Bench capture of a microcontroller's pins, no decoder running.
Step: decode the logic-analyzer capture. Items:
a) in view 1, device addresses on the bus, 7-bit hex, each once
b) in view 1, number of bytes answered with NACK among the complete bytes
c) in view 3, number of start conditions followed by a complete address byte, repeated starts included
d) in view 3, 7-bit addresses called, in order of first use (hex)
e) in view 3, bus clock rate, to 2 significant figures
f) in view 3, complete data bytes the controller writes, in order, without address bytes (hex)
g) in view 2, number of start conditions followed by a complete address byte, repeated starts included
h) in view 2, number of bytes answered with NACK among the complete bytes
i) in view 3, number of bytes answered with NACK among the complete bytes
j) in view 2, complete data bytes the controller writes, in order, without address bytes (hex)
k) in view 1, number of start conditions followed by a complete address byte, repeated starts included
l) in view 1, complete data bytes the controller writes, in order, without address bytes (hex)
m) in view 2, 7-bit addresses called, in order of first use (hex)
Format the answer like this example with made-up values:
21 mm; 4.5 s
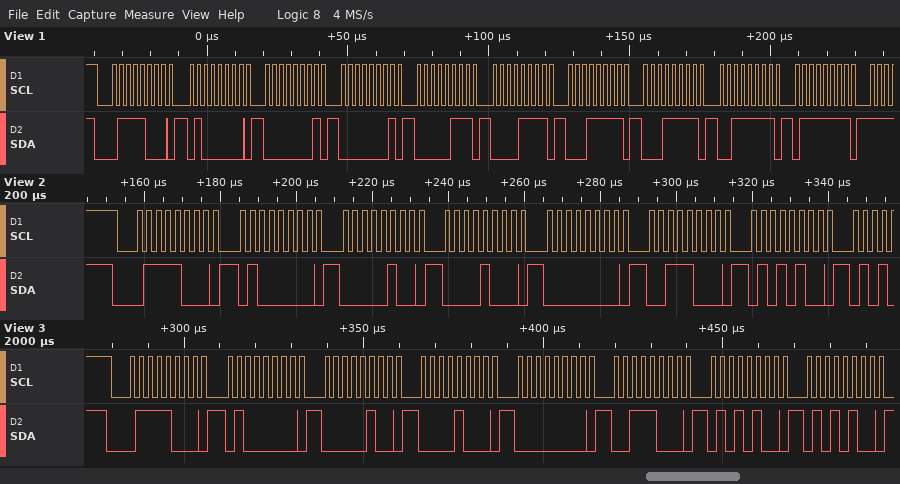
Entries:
0x3C; 0; 1; 0x3C; 400 kHz; 40 04 08 00 38 54 54; 1; 0; 0; 40 04 08 00 38 54; 1; 40 01 01 07 0F 1F 1F 3F 7F; 0x3C
